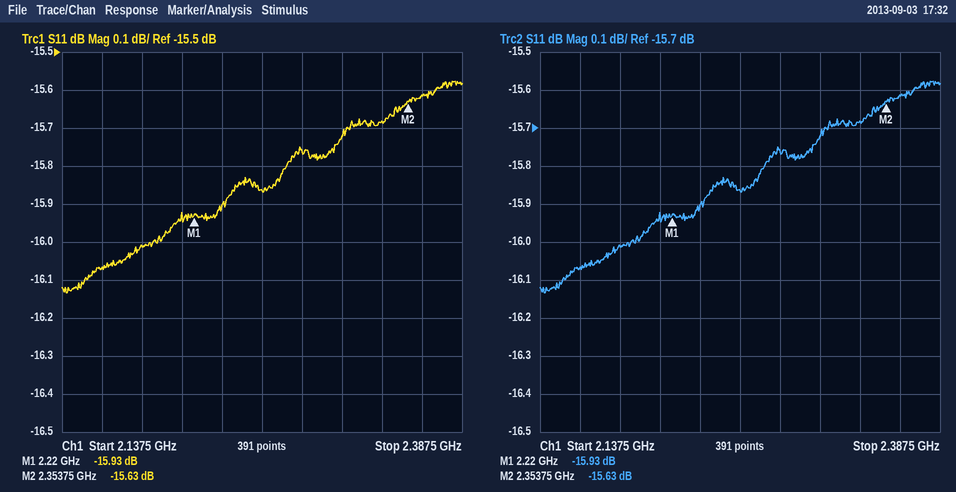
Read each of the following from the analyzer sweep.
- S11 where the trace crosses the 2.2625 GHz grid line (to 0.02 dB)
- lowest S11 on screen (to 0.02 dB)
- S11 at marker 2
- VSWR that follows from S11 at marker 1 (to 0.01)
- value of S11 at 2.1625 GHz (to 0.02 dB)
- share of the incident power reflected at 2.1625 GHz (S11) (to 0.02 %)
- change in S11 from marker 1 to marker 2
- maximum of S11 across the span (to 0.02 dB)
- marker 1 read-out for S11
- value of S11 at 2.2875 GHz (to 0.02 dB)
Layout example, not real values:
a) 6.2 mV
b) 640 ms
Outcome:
a) -15.86 dB
b) -16.14 dB
c) -15.63 dB
d) 1.38
e) -16.06 dB
f) 2.48 %
g) 0.30 dB
h) -15.58 dB
i) -15.93 dB
j) -15.76 dB
